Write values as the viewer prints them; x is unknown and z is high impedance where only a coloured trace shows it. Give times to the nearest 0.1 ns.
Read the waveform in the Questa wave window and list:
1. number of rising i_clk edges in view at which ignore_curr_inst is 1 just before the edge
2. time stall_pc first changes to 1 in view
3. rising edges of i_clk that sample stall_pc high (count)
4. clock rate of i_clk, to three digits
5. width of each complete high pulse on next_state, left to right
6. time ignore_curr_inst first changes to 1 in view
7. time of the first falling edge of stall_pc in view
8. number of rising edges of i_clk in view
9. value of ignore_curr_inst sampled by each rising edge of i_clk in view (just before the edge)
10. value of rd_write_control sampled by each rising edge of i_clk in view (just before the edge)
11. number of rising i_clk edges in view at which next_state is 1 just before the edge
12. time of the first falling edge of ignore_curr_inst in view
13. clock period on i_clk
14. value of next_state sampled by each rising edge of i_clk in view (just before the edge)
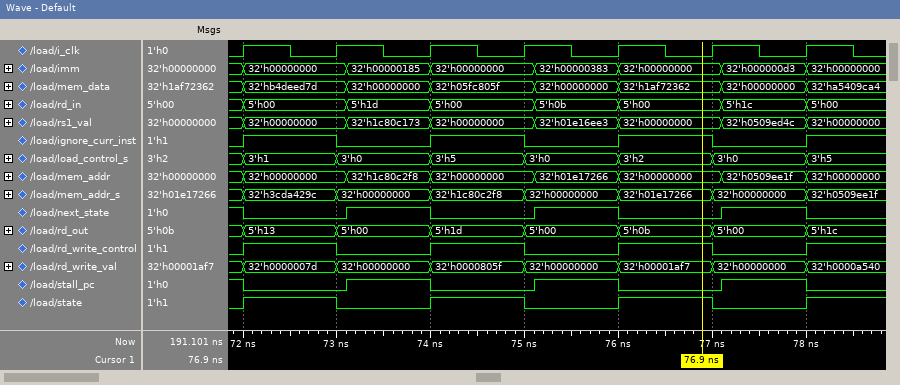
3
73.1 ns
4
1.00 GHz
0.9 ns, 0.9 ns, 0.9 ns
72 ns
72 ns
7
0 1 0 1 0 1 0
0 1 0 1 0 1 0
4
73 ns
1 ns
1 0 1 0 1 0 1
